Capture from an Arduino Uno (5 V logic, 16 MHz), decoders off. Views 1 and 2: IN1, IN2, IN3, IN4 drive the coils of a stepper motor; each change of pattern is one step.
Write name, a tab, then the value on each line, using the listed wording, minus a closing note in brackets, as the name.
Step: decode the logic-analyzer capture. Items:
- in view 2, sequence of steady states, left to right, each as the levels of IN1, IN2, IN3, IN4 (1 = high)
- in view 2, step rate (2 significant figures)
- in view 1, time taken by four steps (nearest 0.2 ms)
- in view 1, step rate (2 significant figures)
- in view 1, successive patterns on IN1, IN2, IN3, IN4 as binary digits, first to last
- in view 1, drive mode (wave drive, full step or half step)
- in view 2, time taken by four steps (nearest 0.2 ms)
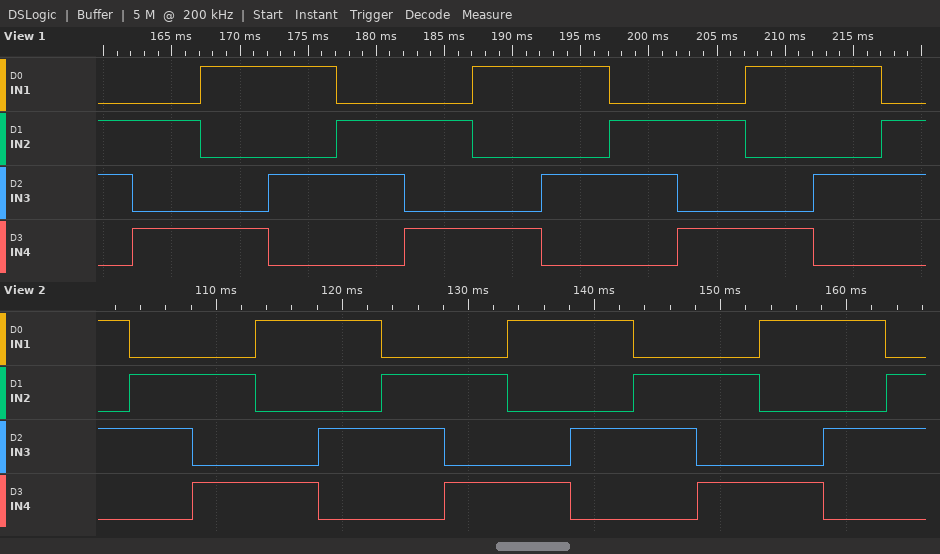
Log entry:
in view 2, sequence of steady states, left to right, each as the levels of IN1, IN2, IN3, IN4	1010 0110 0101 1001 1010 0110 0101 1001 1010 0110 0101 1001 1010 0110
in view 2, step rate	200 steps/s
in view 1, time taken by four steps	20.0 ms
in view 1, step rate	200 steps/s
in view 1, successive patterns on IN1, IN2, IN3, IN4 as binary digits, first to last	0110 0101 1001 1010 0110 0101 1001 1010 0110 0101 1001 1010 0110
in view 1, drive mode	full step
in view 2, time taken by four steps	20.0 ms
